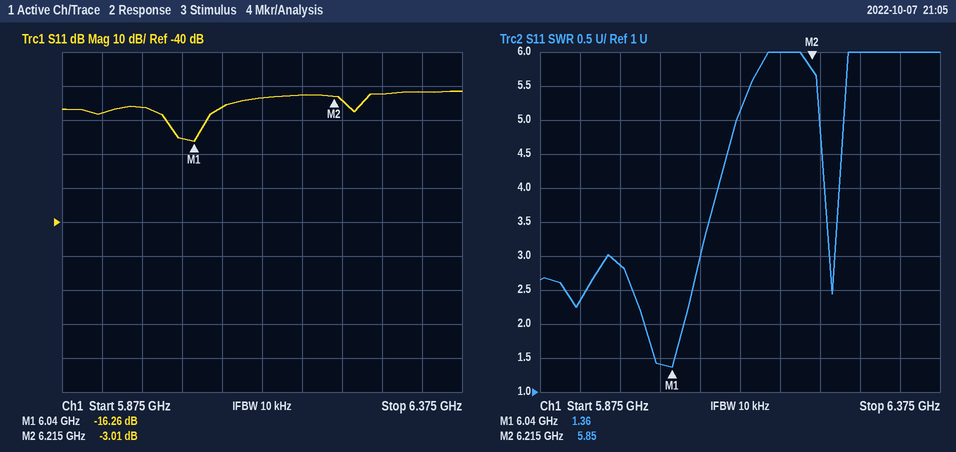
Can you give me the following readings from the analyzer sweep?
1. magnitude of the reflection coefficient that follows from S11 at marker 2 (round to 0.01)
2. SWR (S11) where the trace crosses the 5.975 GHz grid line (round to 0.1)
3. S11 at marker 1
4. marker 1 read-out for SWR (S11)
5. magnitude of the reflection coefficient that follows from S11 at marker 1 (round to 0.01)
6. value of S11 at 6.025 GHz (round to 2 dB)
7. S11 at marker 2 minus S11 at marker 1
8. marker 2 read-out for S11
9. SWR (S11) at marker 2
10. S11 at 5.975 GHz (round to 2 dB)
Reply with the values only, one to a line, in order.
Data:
0.71
2.9
-16.26 dB
1.36
0.15
-16 dB
13.25 dB
-3.01 dB
5.85
-6 dB
